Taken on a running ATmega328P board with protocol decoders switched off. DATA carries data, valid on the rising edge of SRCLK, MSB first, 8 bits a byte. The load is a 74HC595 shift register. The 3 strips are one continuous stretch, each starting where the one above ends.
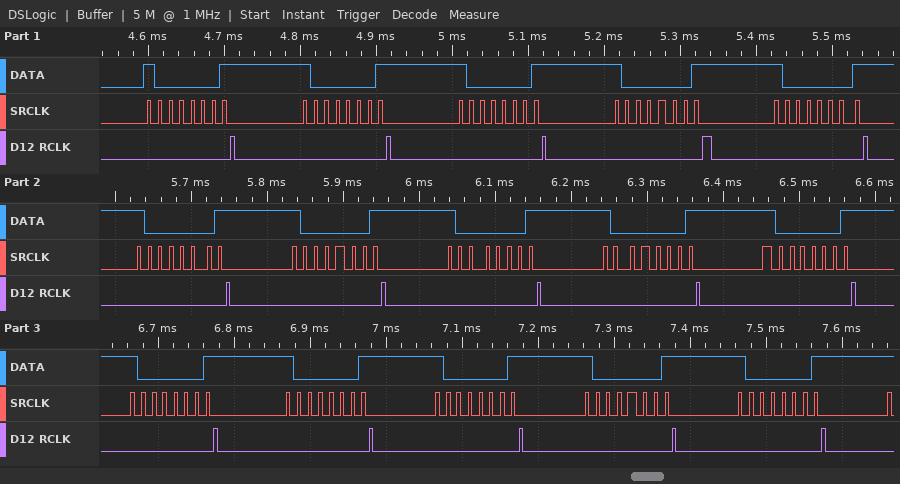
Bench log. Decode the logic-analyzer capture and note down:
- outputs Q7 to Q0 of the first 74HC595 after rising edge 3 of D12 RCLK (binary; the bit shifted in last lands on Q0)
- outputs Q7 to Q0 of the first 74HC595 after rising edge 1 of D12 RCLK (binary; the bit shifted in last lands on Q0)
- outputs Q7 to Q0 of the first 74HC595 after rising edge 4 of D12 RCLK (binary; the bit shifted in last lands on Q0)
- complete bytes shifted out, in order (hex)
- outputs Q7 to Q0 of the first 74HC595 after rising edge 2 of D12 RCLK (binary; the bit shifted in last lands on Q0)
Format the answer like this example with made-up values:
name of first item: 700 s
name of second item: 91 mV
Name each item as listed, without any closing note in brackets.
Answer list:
outputs Q7 to Q0 of the first 74HC595 after rising edge 3 of D12 RCLK: 10000001
outputs Q7 to Q0 of the first 74HC595 after rising edge 1 of D12 RCLK: 10000001
outputs Q7 to Q0 of the first 74HC595 after rising edge 4 of D12 RCLK: 10000001
complete bytes shifted out, in order: 81 81 81 81 81 81 81 81 81 81 81 81 81 81 81
outputs Q7 to Q0 of the first 74HC595 after rising edge 2 of D12 RCLK: 10000001
